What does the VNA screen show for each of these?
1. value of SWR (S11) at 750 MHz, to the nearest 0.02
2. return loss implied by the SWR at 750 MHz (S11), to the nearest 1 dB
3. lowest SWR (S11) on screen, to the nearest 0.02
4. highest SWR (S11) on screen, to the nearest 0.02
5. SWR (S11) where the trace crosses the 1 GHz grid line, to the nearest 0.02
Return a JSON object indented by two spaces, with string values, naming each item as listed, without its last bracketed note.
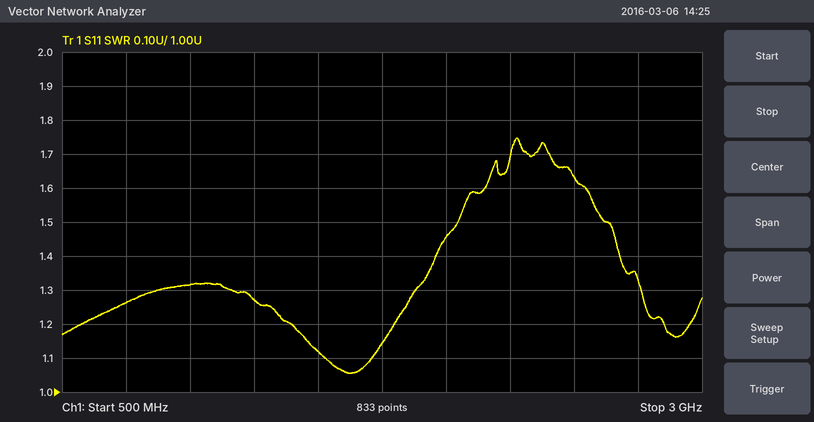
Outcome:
{
  "value of SWR (S11) at 750 MHz, to the nearest 0.02": "1.26",
  "return loss implied by the SWR at 750 MHz (S11), to the nearest 1 dB": "19 dB",
  "lowest SWR (S11) on screen, to the nearest 0.02": "1.06",
  "highest SWR (S11) on screen, to the nearest 0.02": "1.74",
  "SWR (S11) where the trace crosses the 1 GHz grid line, to the nearest 0.02": "1.32"
}
